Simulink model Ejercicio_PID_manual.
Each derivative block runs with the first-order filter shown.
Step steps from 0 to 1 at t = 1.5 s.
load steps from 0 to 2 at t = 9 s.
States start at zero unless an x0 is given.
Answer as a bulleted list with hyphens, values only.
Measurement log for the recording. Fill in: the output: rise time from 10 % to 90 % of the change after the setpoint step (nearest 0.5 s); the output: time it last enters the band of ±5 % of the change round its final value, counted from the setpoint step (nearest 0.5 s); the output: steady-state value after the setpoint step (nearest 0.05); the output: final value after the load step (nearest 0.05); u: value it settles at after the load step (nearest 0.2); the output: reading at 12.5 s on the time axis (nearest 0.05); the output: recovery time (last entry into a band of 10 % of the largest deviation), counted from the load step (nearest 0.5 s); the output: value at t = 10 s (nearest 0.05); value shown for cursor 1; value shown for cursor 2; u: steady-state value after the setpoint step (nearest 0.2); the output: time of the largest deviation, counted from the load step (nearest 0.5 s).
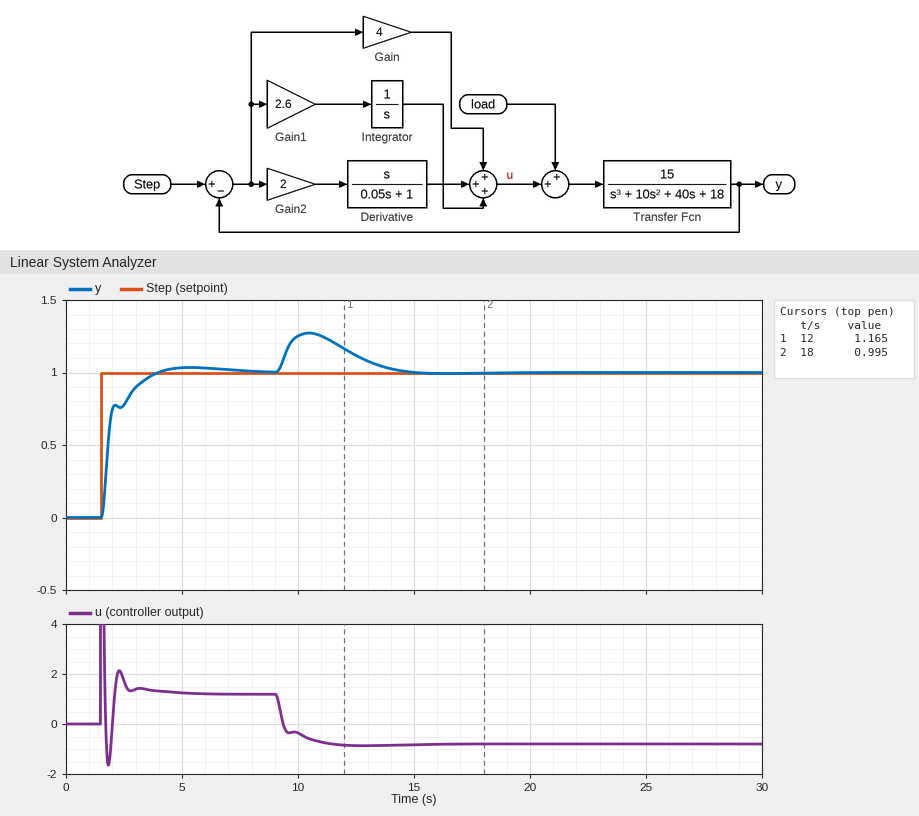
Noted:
- 1.5 s
- 2.0 s
- 1.00
- 1.00
- -0.8
- 1.10
- 5.0 s
- 1.25
- 1.165
- 0.995
- 1.2
- 1.5 s
